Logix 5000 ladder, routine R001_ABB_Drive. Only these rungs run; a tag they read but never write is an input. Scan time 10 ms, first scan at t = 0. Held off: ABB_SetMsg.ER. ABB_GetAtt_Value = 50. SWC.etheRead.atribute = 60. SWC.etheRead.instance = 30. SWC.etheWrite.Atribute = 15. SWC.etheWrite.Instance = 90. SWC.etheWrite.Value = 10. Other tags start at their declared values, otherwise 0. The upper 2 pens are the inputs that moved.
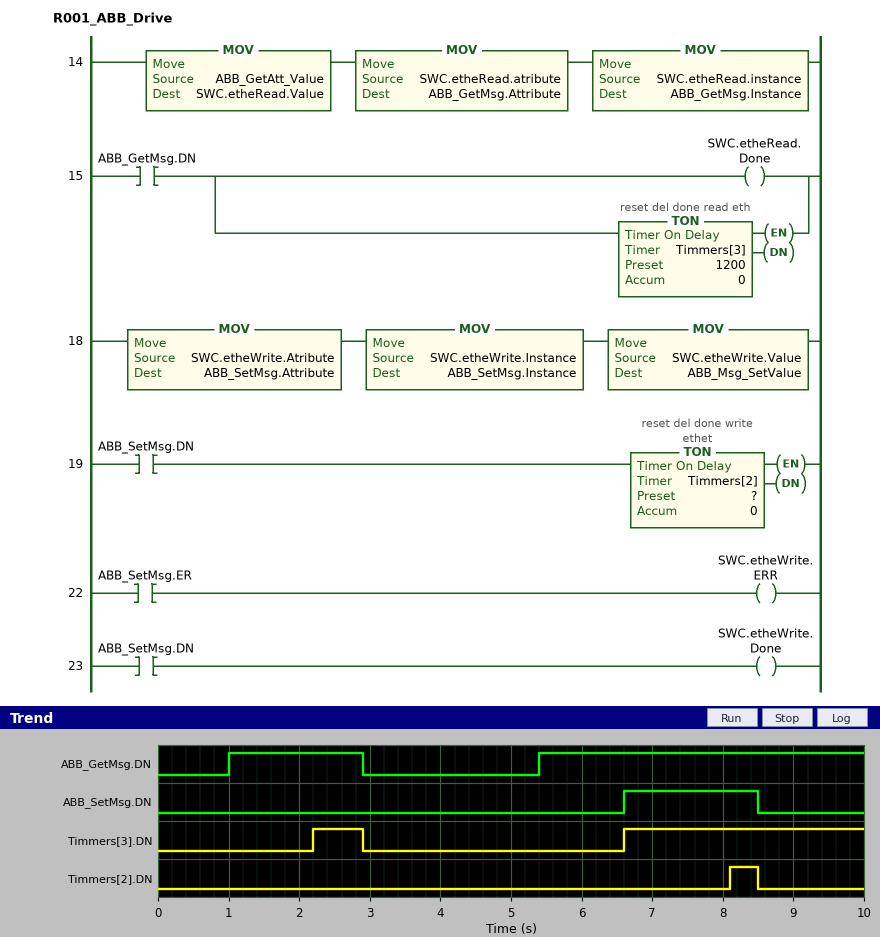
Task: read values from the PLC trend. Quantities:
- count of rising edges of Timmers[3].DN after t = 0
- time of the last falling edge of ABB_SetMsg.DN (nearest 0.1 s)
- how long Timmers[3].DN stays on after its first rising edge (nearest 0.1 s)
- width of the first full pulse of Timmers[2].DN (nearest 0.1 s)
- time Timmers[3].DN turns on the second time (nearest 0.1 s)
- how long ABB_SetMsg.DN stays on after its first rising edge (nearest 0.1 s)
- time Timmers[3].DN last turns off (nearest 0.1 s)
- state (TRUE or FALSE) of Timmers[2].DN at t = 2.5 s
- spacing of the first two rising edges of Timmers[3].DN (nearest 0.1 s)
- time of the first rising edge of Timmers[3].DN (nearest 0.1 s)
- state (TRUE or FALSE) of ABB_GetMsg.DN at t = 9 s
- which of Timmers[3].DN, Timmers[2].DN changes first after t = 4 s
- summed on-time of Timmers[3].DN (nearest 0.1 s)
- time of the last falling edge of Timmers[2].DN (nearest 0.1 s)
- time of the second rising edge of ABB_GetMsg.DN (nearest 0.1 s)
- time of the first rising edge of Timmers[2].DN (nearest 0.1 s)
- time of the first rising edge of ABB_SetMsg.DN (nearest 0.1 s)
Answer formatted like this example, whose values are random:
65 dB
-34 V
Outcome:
2
8.5 s
0.7 s
0.4 s
6.6 s
1.9 s
2.9 s
FALSE
4.4 s
2.2 s
TRUE
Timmers[3].DN
4.1 s
8.5 s
5.4 s
8.1 s
6.6 s
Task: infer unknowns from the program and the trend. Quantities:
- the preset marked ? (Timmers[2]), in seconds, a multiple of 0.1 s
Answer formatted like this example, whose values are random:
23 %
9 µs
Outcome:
1.5 s
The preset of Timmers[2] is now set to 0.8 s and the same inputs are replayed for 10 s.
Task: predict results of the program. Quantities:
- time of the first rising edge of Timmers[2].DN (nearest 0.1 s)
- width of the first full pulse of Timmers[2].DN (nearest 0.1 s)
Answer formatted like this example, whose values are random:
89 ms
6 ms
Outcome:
7.4 s
1.1 s
